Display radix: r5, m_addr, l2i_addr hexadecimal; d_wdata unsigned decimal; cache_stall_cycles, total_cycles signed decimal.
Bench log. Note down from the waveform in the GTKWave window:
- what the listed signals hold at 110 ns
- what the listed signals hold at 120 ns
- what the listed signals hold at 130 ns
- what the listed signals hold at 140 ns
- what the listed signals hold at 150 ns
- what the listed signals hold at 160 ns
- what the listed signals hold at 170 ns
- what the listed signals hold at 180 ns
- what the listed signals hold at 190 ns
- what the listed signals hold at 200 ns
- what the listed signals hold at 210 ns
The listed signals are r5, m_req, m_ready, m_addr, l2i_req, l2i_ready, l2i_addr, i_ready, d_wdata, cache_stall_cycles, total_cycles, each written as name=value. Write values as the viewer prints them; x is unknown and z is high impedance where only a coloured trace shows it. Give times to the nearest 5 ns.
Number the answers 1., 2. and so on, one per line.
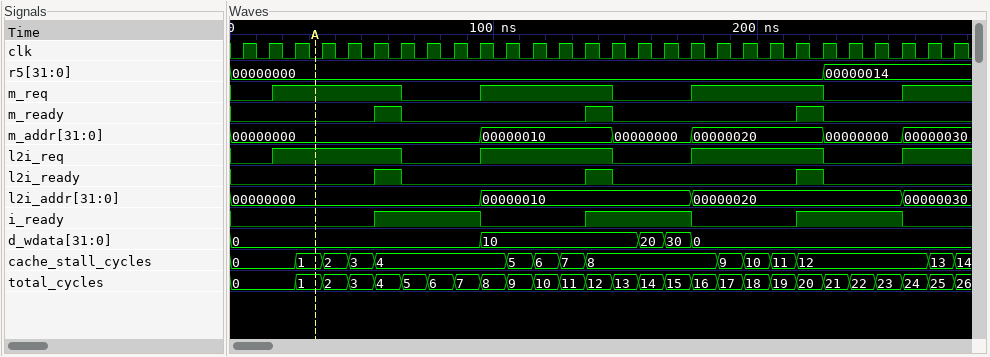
1. r5=00000000, m_req=1, m_ready=0, m_addr=00000010, l2i_req=1, l2i_ready=0, l2i_addr=00000010, i_ready=0, d_wdata=10, cache_stall_cycles=5, total_cycles=9
2. r5=00000000, m_req=1, m_ready=0, m_addr=00000010, l2i_req=1, l2i_ready=0, l2i_addr=00000010, i_ready=0, d_wdata=10, cache_stall_cycles=6, total_cycles=10
3. r5=00000000, m_req=1, m_ready=0, m_addr=00000010, l2i_req=1, l2i_ready=0, l2i_addr=00000010, i_ready=0, d_wdata=10, cache_stall_cycles=7, total_cycles=11
4. r5=00000000, m_req=1, m_ready=1, m_addr=00000010, l2i_req=1, l2i_ready=1, l2i_addr=00000010, i_ready=1, d_wdata=10, cache_stall_cycles=8, total_cycles=12
5. r5=00000000, m_req=0, m_ready=0, m_addr=00000000, l2i_req=0, l2i_ready=0, l2i_addr=00000010, i_ready=1, d_wdata=10, cache_stall_cycles=8, total_cycles=13
6. r5=00000000, m_req=0, m_ready=0, m_addr=00000000, l2i_req=0, l2i_ready=0, l2i_addr=00000010, i_ready=1, d_wdata=20, cache_stall_cycles=8, total_cycles=14
7. r5=00000000, m_req=0, m_ready=0, m_addr=00000000, l2i_req=0, l2i_ready=0, l2i_addr=00000010, i_ready=1, d_wdata=30, cache_stall_cycles=8, total_cycles=15
8. r5=00000000, m_req=1, m_ready=0, m_addr=00000020, l2i_req=1, l2i_ready=0, l2i_addr=00000020, i_ready=0, d_wdata=0, cache_stall_cycles=8, total_cycles=16
9. r5=00000000, m_req=1, m_ready=0, m_addr=00000020, l2i_req=1, l2i_ready=0, l2i_addr=00000020, i_ready=0, d_wdata=0, cache_stall_cycles=9, total_cycles=17
10. r5=00000000, m_req=1, m_ready=0, m_addr=00000020, l2i_req=1, l2i_ready=0, l2i_addr=00000020, i_ready=0, d_wdata=0, cache_stall_cycles=10, total_cycles=18
11. r5=00000000, m_req=1, m_ready=0, m_addr=00000020, l2i_req=1, l2i_ready=0, l2i_addr=00000020, i_ready=0, d_wdata=0, cache_stall_cycles=11, total_cycles=19
